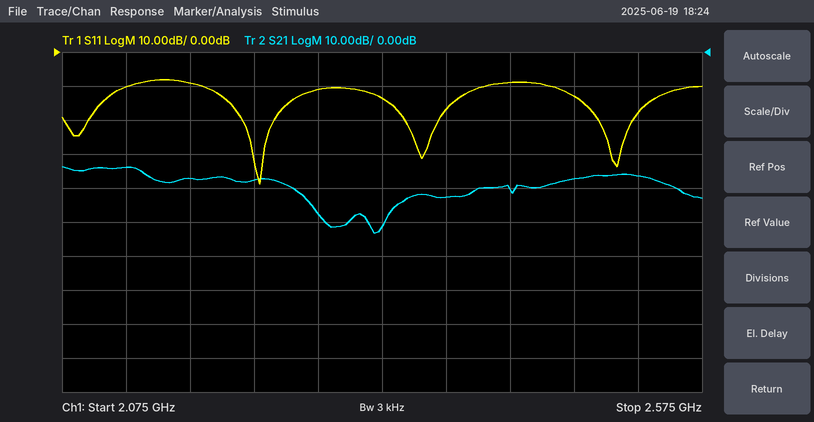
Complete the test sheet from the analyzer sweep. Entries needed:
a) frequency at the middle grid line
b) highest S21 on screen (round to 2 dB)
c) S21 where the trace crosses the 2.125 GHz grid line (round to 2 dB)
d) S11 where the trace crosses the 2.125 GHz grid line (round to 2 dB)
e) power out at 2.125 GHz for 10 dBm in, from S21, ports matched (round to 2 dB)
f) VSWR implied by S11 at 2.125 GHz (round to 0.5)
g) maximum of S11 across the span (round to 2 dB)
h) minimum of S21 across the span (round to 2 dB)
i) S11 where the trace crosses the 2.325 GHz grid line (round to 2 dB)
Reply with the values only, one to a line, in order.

2.325 GHz
-34 dB
-34 dB
-10 dB
-24 dBm
2.0
-8 dB
-54 dB
-14 dB
